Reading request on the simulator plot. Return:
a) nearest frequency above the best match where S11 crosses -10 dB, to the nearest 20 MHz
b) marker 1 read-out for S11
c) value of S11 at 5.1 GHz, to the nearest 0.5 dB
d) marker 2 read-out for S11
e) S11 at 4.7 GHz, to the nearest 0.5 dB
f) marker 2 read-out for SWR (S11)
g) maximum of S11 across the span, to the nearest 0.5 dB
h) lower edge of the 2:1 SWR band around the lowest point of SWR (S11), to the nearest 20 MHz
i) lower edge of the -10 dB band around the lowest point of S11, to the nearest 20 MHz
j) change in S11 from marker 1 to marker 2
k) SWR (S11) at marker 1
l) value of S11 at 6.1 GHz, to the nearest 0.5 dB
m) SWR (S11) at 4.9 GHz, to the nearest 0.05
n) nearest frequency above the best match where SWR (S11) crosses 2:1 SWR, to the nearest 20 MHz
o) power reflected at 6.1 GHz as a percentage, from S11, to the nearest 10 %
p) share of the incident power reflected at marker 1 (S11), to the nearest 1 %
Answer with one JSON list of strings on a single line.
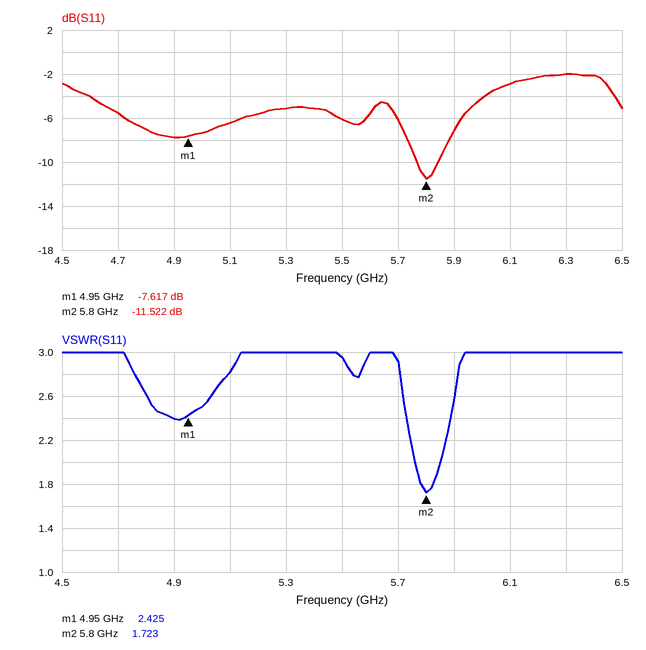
["5.84 GHz", "-7.617 dB", "-6.5 dB", "-11.522 dB", "-5.5 dB", "1.723", "-2.0 dB", "5.76 GHz", "5.76 GHz", "-3.905 dB", "2.425", "-3.0 dB", "2.40", "5.86 GHz", "50 %", "17 %"]
